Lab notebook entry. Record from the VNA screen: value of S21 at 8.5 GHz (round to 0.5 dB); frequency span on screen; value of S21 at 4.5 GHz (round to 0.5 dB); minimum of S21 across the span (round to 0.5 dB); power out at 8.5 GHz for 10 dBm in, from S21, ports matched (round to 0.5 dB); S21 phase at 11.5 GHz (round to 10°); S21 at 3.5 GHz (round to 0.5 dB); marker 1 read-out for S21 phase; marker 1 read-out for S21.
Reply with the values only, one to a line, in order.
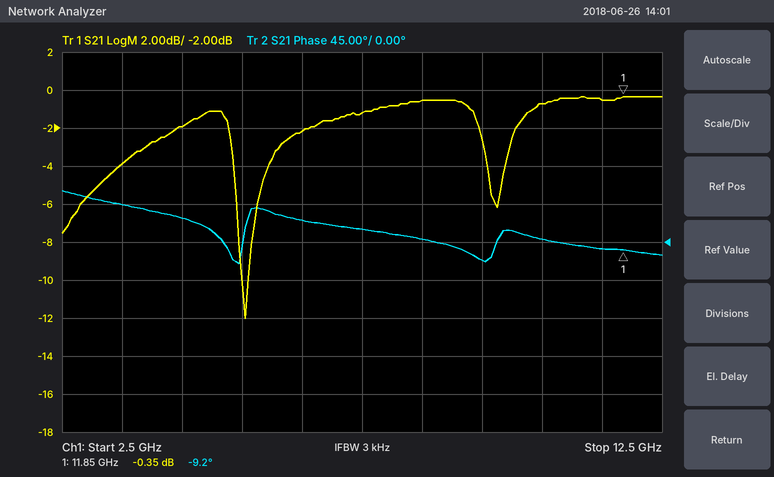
-0.5 dB
10 GHz
-2.0 dB
-12.0 dB
9.5 dBm
-10°
-4.0 dB
-9.2°
-0.35 dB
